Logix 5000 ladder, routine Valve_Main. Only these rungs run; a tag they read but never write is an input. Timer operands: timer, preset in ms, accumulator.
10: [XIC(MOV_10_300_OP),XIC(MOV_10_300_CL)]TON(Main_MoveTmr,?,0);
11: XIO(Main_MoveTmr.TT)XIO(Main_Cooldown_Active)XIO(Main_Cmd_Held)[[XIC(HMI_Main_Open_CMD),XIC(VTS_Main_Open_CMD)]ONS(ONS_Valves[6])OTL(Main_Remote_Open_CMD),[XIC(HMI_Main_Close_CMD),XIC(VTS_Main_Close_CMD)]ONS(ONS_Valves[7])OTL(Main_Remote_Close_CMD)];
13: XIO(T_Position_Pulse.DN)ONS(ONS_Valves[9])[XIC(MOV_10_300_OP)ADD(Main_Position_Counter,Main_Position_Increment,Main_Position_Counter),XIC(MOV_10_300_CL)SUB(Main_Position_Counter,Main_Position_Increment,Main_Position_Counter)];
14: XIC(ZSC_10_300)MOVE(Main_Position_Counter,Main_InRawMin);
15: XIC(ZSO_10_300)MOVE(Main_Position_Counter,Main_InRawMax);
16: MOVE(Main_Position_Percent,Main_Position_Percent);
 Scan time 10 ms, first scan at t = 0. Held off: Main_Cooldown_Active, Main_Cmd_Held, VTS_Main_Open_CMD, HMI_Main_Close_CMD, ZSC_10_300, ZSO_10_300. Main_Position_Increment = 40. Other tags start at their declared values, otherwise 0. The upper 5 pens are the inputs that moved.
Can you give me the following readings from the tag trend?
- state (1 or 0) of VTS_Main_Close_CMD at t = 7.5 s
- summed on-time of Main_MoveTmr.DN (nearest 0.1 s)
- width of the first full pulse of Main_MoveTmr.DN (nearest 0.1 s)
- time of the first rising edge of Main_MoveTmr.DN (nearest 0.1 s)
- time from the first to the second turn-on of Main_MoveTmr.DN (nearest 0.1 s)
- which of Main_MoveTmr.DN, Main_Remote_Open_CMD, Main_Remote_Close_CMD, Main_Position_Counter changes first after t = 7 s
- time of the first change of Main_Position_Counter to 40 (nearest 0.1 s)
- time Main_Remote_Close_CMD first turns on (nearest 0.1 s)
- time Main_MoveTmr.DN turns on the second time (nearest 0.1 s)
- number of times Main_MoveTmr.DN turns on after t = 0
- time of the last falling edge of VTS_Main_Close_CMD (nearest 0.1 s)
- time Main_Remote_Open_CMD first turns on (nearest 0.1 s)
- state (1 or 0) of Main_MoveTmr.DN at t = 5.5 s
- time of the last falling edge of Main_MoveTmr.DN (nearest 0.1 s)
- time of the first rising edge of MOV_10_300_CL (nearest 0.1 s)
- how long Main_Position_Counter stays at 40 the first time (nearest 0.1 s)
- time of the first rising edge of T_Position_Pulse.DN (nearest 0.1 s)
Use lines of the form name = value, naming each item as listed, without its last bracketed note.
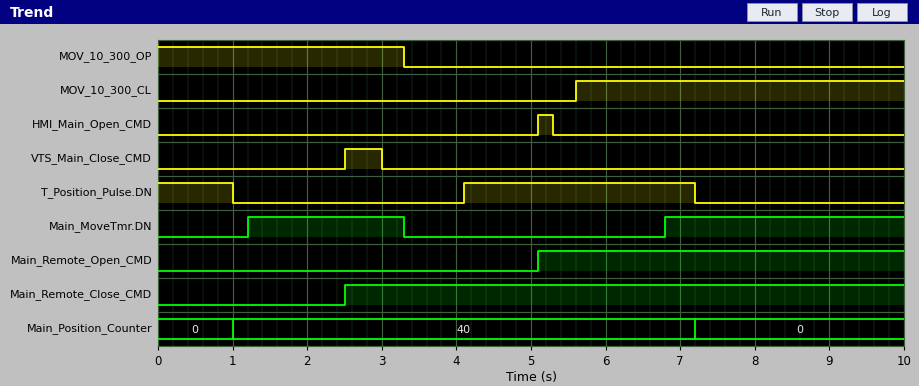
state (1 or 0) of VTS_Main_Close_CMD at t = 7.5 s = 0
summed on-time of Main_MoveTmr.DN = 5.3 s
width of the first full pulse of Main_MoveTmr.DN = 2.1 s
time of the first rising edge of Main_MoveTmr.DN = 1.2 s
time from the first to the second turn-on of Main_MoveTmr.DN = 5.6 s
which of Main_MoveTmr.DN, Main_Remote_Open_CMD, Main_Remote_Close_CMD, Main_Position_Counter changes first after t = 7 s = Main_Position_Counter
time of the first change of Main_Position_Counter to 40 = 1.0 s
time Main_Remote_Close_CMD first turns on = 2.5 s
time Main_MoveTmr.DN turns on the second time = 6.8 s
number of times Main_MoveTmr.DN turns on after t = 0 = 2
time of the last falling edge of VTS_Main_Close_CMD = 3.0 s
time Main_Remote_Open_CMD first turns on = 5.1 s
state (1 or 0) of Main_MoveTmr.DN at t = 5.5 s = 0
time of the last falling edge of Main_MoveTmr.DN = 3.3 s
time of the first rising edge of MOV_10_300_CL = 5.6 s
how long Main_Position_Counter stays at 40 the first time = 6.2 s
time of the first rising edge of T_Position_Pulse.DN = 4.1 s
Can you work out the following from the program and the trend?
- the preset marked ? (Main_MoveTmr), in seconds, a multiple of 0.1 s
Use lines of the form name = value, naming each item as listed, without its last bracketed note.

the preset marked ? (Main_MoveTmr), in seconds, a multiple of 0.1 s = 1.2 s
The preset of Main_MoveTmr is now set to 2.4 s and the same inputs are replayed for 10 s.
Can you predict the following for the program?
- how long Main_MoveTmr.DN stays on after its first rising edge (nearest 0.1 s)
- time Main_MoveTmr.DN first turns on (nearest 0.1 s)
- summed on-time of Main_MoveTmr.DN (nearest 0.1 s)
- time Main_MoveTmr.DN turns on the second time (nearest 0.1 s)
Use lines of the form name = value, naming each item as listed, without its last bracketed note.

how long Main_MoveTmr.DN stays on after its first rising edge = 0.9 s
time Main_MoveTmr.DN first turns on = 2.4 s
summed on-time of Main_MoveTmr.DN = 2.9 s
time Main_MoveTmr.DN turns on the second time = 8.0 s
